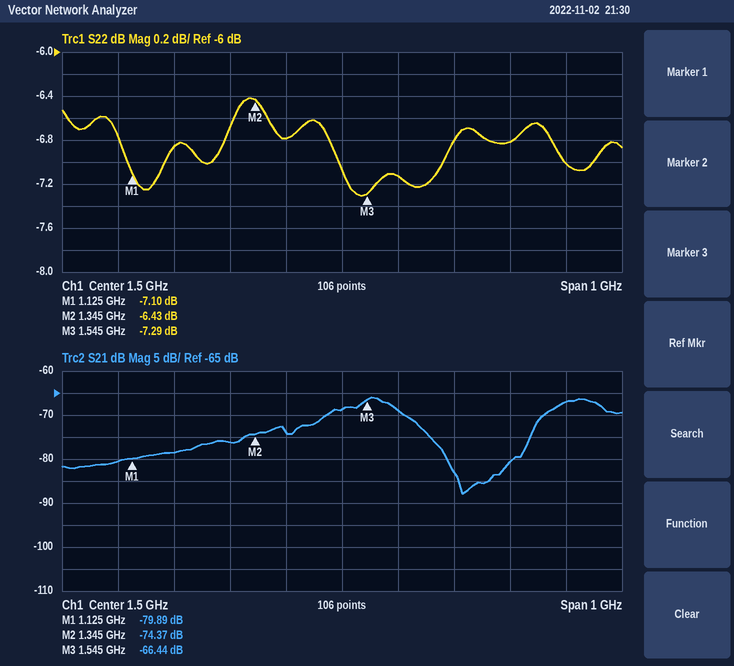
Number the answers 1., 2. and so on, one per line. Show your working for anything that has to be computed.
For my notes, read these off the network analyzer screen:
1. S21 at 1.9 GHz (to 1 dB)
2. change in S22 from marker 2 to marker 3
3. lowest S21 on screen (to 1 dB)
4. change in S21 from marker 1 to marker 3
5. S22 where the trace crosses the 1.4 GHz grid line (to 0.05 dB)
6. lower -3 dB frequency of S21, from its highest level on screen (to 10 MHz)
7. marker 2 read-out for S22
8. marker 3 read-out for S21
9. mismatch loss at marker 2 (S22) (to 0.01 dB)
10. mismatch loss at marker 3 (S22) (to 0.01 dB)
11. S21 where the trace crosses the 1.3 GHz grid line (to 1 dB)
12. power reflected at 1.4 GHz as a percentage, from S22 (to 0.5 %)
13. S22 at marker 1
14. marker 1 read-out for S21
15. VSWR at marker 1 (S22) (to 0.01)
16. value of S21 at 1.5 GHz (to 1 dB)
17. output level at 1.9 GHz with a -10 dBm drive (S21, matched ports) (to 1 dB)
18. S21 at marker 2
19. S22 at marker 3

1. -67 dB
2. -7.29 − (-6.43) = -0.86 dB
3. -88 dB
4. -66.44 − (-79.89) = 13.45 dB
5. -6.80 dB
6. 1.48 GHz
7. -6.43 dB
8. -66.44 dB
9. −10 log10(1 − 10^(-6.43/10)) ≈ 1.12 dB
10. −10 log10(1 − 10^(-7.29/10)) ≈ 0.90 dB
11. -76 dB
12. 10^(-6.8/10) ≈ 20.9 %, so 21.0 % to the nearest 0.5 %
13. -7.10 dB
14. -79.89 dB
15. (1 + 0.4416)/(1 − 0.4416) ≈ 2.58
16. -69 dB
17. -10 dBm + (-67 dB) = -77 dBm
18. -74.37 dB
19. -7.29 dB
